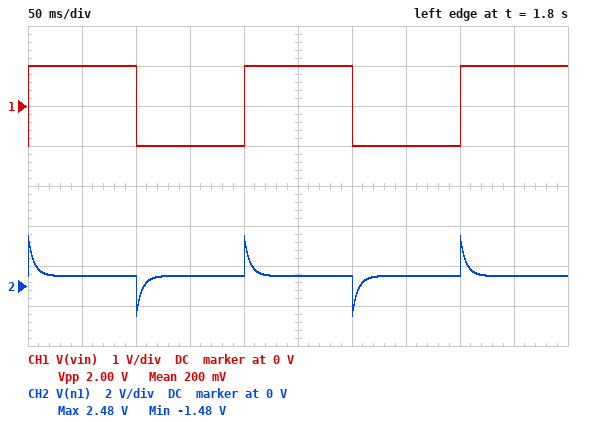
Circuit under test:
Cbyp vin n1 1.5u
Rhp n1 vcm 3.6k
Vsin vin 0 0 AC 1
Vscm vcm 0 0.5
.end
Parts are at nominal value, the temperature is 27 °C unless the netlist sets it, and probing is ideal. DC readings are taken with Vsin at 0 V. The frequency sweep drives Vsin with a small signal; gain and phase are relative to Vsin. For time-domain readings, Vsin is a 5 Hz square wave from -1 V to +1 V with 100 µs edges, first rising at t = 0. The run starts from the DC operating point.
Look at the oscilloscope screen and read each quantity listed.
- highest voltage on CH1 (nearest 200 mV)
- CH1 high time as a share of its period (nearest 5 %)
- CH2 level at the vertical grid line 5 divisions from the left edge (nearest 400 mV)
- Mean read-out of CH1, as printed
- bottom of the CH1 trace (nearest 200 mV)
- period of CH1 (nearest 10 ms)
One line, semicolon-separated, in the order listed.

1.0 V; 50 %; 400 mV; 200 mV; -1.0 V; 200 ms
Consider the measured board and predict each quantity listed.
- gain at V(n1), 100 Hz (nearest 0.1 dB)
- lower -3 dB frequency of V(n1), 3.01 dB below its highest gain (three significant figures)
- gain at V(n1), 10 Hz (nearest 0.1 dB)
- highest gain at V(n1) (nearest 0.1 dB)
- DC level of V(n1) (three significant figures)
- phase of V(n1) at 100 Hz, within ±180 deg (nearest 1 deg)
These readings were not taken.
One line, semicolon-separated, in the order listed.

-0.4 dB; 29.5 Hz; -9.9 dB; 0 dB; 500 mV; 16 deg
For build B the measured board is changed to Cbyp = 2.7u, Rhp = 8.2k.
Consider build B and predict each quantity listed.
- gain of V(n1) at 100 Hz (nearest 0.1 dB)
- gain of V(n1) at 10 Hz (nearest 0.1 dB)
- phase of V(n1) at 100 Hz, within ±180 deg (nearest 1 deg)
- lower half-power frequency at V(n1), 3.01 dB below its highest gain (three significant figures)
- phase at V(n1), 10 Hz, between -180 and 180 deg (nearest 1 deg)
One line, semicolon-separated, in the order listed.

0 dB; -1.8 dB; 4 deg; 7.19 Hz; 36 deg
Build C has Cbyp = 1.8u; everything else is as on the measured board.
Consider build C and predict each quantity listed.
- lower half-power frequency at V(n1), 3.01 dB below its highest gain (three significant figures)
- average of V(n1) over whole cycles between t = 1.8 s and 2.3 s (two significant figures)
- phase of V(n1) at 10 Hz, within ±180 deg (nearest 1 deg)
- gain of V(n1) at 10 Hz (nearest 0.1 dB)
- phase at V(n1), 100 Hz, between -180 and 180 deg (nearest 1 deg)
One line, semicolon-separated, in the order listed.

24.6 Hz; 500 mV; 68 deg; -8.5 dB; 14 deg
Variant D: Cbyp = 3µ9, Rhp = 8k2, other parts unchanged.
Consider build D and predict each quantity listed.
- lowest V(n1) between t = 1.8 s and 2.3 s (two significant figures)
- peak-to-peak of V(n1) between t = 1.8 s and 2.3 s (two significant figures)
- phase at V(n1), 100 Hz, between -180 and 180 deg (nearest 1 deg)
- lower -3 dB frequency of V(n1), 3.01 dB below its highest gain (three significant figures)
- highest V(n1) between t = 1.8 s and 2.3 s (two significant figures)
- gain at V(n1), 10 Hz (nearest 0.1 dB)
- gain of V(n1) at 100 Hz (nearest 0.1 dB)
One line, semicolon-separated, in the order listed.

-1.4 V; 3.8 V; 3 deg; 4.98 Hz; 2.4 V; -1.0 dB; 0 dB
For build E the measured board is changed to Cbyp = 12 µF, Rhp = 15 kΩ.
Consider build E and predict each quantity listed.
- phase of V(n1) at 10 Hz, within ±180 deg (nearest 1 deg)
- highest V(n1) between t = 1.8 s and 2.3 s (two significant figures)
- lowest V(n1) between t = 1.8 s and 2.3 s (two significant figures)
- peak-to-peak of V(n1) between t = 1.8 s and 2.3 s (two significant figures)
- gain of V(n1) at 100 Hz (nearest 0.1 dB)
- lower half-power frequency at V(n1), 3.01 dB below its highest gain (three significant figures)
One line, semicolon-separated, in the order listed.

5 deg; 1.8 V; -770 mV; 2.5 V; 0 dB; 884 mHz
